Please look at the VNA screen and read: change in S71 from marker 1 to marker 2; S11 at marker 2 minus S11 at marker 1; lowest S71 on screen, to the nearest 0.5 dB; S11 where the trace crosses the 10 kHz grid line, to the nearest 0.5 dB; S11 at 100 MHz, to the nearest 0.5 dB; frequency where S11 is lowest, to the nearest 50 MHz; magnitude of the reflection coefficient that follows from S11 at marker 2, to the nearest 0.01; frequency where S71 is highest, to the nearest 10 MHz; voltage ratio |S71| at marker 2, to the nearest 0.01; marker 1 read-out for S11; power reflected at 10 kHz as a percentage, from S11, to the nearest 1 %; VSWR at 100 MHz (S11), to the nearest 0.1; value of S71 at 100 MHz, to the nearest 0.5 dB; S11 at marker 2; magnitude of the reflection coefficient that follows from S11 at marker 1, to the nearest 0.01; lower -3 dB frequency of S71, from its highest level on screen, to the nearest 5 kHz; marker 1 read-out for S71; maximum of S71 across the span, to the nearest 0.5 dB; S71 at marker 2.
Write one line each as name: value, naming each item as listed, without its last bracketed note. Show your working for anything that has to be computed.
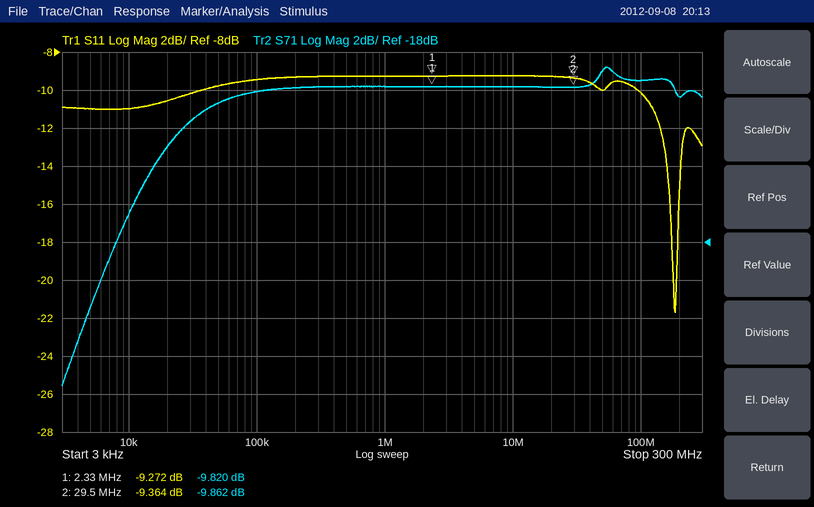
change in S71 from marker 1 to marker 2: -9.862 − (-9.82) = -0.042 dB
S11 at marker 2 minus S11 at marker 1: -9.364 − (-9.272) = -0.092 dB
lowest S71 on screen, to the nearest 0.5 dB: -25.5 dB
S11 where the trace crosses the 10 kHz grid line, to the nearest 0.5 dB: -11.0 dB
S11 at 100 MHz, to the nearest 0.5 dB: -10.0 dB
frequency where S11 is lowest, to the nearest 50 MHz: 200 MHz
magnitude of the reflection coefficient that follows from S11 at marker 2, to the nearest 0.01: 10^(-9.364/20) ≈ 0.34
frequency where S71 is highest, to the nearest 10 MHz: 50 MHz
voltage ratio |S71| at marker 2, to the nearest 0.01: 10^(-9.862/20) ≈ 0.32
marker 1 read-out for S11: -9.272 dB
power reflected at 10 kHz as a percentage, from S11, to the nearest 1 %: 10^(-11/10) ≈ 8 %
VSWR at 100 MHz (S11), to the nearest 0.1: |Γ| = 10^(-10/20) = 0.3162; VSWR = (1 + 0.3162)/(1 − 0.3162) ≈ 1.9
value of S71 at 100 MHz, to the nearest 0.5 dB: -9.5 dB
S11 at marker 2: -9.364 dB
magnitude of the reflection coefficient that follows from S11 at marker 1, to the nearest 0.01: 10^(-9.272/20) ≈ 0.34
lower -3 dB frequency of S71, from its highest level on screen, to the nearest 5 kHz: 30 kHz
marker 1 read-out for S71: -9.820 dB
maximum of S71 across the span, to the nearest 0.5 dB: -9.0 dB
S71 at marker 2: -9.862 dB
